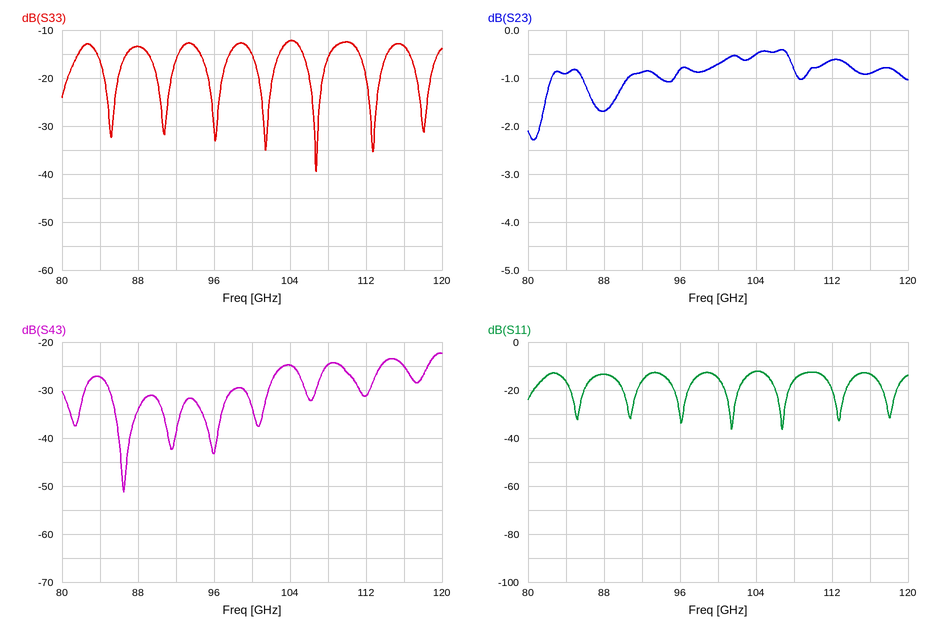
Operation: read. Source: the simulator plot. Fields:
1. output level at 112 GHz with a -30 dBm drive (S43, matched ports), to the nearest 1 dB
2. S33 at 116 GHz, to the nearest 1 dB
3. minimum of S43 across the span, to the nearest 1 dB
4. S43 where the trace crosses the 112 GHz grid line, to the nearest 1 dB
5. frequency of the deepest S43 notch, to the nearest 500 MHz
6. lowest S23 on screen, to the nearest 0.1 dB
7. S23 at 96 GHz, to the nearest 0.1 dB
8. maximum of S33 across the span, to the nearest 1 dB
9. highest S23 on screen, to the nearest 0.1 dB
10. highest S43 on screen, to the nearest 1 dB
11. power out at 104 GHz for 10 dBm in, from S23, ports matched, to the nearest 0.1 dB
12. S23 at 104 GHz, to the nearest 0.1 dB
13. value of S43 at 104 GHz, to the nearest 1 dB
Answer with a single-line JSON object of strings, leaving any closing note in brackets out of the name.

{"output level at 112 GHz with a -30 dBm drive (S43, matched ports), to the nearest 1 dB": "-61 dBm", "S33 at 116 GHz, to the nearest 1 dB": "-13 dB", "minimum of S43 across the span, to the nearest 1 dB": "-51 dB", "S43 where the trace crosses the 112 GHz grid line, to the nearest 1 dB": "-31 dB", "frequency of the deepest S43 notch, to the nearest 500 MHz": "86.5 GHz", "lowest S23 on screen, to the nearest 0.1 dB": "-2.3 dB", "S23 at 96 GHz, to the nearest 0.1 dB": "-0.8 dB", "maximum of S33 across the span, to the nearest 1 dB": "-12 dB", "highest S23 on screen, to the nearest 0.1 dB": "-0.4 dB", "highest S43 on screen, to the nearest 1 dB": "-22 dB", "power out at 104 GHz for 10 dBm in, from S23, ports matched, to the nearest 0.1 dB": "9.5 dBm", "S23 at 104 GHz, to the nearest 0.1 dB": "-0.5 dB", "value of S43 at 104 GHz, to the nearest 1 dB": "-25 dB"}
